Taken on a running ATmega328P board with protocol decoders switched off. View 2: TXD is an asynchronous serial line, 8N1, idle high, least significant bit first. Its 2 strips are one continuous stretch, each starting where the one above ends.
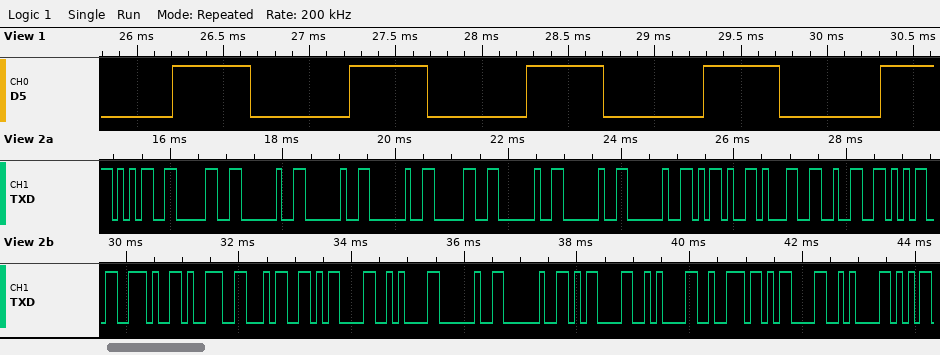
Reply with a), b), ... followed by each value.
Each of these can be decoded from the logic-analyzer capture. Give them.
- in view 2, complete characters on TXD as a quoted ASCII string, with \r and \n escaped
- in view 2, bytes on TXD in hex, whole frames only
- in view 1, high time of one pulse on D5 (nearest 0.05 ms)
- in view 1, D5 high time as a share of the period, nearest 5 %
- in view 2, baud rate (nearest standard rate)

a) "50   0   -125.94\r\n  \r\nr\r\n"
b) 35 30 20 20 20 30 20 20 20 2D 31 32 35 2E 39 34 0D 0A 20 20 0D 0A 72 0D 0A
c) 0.45 ms
d) 45 %
e) 9600 baud
